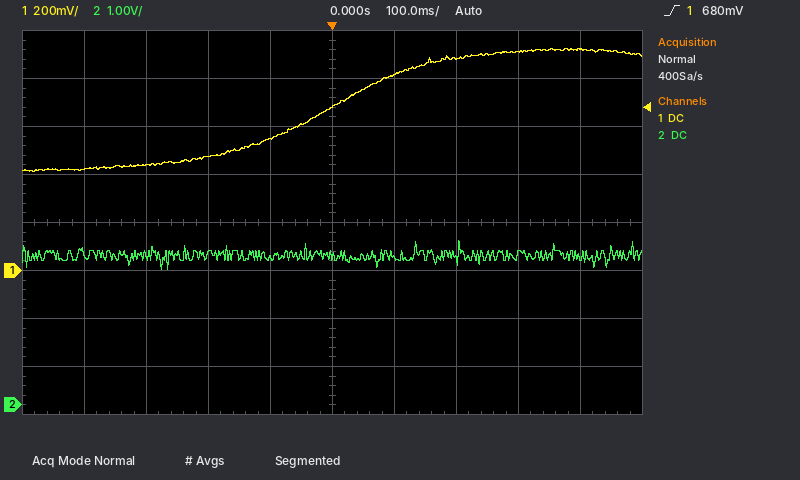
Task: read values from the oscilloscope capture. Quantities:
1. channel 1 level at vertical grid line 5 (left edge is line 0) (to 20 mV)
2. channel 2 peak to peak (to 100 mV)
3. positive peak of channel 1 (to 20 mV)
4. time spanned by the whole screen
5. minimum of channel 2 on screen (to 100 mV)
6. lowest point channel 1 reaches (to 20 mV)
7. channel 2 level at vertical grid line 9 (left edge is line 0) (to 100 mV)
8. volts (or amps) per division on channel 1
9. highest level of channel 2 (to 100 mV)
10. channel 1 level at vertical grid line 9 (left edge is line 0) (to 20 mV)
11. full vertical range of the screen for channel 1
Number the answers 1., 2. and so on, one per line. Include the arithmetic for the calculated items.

1. 680 mV
2. 3.4 V − (2.8 V) = 600 mV
3. 920 mV
4. 1 s
5. 2.8 V
6. 420 mV
7. 3.1 V
8. 200 mV
9. 3.4 V
10. 920 mV
11. 1.6 V
